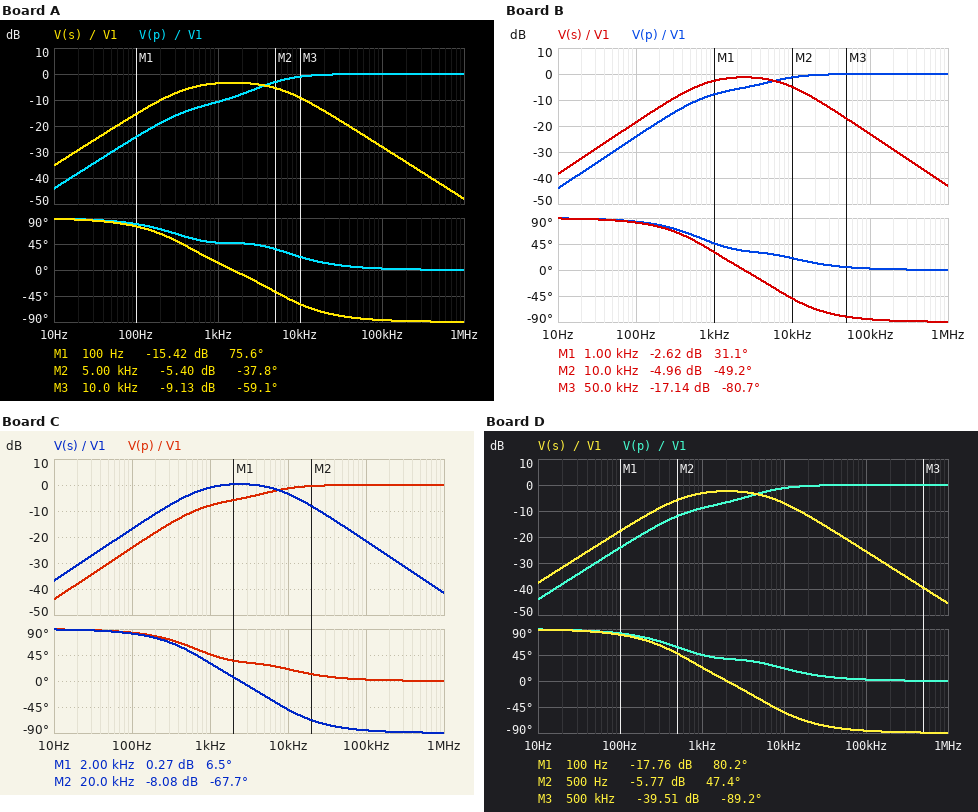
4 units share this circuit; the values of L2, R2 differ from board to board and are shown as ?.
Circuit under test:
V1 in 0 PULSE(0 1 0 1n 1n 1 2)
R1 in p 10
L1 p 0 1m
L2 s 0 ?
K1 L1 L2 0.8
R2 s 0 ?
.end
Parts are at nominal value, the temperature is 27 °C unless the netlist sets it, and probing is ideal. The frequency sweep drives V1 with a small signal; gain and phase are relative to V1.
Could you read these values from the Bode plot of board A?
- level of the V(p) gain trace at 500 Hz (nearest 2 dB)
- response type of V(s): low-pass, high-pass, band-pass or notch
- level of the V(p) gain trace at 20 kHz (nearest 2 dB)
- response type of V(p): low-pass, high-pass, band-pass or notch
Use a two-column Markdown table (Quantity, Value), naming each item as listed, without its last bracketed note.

| Quantity | Value |
|---|---|
| level of the V(p) gain trace at 500 Hz | -14 dB |
| response type of V(s): low-pass, high-pass, band-pass or notch | band-pass |
| level of the V(p) gain trace at 20 kHz | 0 dB |
| response type of V(p): low-pass, high-pass, band-pass or notch | high-pass |
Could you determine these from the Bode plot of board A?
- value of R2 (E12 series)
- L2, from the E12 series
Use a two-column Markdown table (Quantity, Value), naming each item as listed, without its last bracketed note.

| Quantity | Value |
|---|---|
| value of R2 | 39 Ω |
| L2, from the E12 series | 12 mH |
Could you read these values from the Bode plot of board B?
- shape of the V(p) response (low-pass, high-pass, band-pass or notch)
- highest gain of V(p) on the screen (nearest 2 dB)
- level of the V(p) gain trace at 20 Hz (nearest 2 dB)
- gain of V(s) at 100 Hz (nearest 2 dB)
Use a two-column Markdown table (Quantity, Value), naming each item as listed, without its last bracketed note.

| Quantity | Value |
|---|---|
| shape of the V(p) response | high-pass |
| highest gain of V(p) on the screen | 0 dB |
| level of the V(p) gain trace at 20 Hz | -38 dB |
| gain of V(s) at 100 Hz | -18 dB |
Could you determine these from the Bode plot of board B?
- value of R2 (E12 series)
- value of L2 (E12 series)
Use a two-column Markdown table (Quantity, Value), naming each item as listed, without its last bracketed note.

| Quantity | Value |
|---|---|
| value of R2 | 47 Ω |
| value of L2 | 5.6 mH |
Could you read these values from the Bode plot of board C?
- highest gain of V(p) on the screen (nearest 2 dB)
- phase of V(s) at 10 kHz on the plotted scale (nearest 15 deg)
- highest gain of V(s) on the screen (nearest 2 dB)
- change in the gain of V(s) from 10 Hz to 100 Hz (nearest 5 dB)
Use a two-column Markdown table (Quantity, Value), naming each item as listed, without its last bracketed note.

| Quantity | Value |
|---|---|
| highest gain of V(p) on the screen | 0 dB |
| phase of V(s) at 10 kHz on the plotted scale | -45 deg |
| highest gain of V(s) on the screen | 0 dB |
| change in the gain of V(s) from 10 Hz to 100 Hz | 20 dB |
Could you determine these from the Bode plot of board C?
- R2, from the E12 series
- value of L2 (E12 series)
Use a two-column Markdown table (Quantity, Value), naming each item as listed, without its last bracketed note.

| Quantity | Value |
|---|---|
| R2, from the E12 series | 68 Ω |
| value of L2 | 8.2 mH |
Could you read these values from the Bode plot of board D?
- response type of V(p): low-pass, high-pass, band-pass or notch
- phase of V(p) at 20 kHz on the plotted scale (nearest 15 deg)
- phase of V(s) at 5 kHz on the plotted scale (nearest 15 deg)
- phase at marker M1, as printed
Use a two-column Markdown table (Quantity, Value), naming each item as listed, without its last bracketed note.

| Quantity | Value |
|---|---|
| response type of V(p): low-pass, high-pass, band-pass or notch | high-pass |
| phase of V(p) at 20 kHz on the plotted scale | 15 deg |
| phase of V(s) at 5 kHz on the plotted scale | -30 deg |
| phase at marker M1, as printed | 80.2 deg |
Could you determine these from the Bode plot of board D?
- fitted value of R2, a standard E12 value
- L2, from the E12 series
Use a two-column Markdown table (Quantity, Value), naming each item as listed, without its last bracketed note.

| Quantity | Value |
|---|---|
| fitted value of R2, a standard E12 value | 39 Ω |
| L2, from the E12 series | 6.8 mH |
